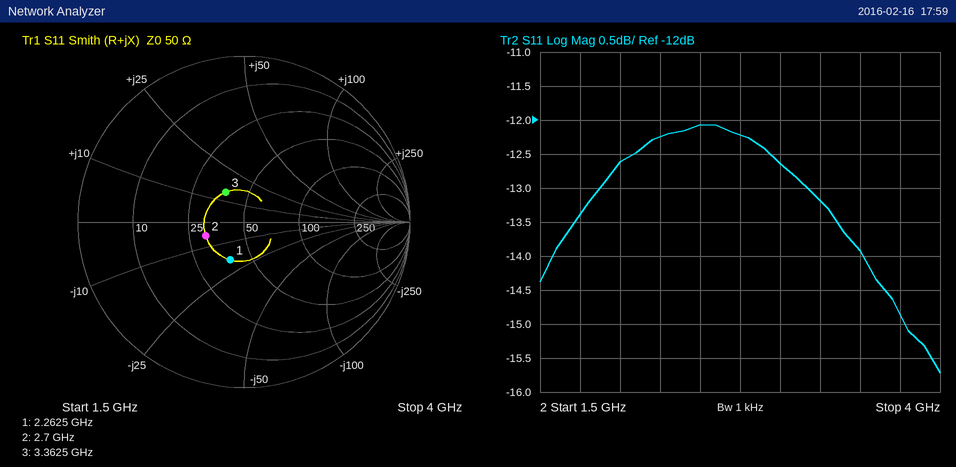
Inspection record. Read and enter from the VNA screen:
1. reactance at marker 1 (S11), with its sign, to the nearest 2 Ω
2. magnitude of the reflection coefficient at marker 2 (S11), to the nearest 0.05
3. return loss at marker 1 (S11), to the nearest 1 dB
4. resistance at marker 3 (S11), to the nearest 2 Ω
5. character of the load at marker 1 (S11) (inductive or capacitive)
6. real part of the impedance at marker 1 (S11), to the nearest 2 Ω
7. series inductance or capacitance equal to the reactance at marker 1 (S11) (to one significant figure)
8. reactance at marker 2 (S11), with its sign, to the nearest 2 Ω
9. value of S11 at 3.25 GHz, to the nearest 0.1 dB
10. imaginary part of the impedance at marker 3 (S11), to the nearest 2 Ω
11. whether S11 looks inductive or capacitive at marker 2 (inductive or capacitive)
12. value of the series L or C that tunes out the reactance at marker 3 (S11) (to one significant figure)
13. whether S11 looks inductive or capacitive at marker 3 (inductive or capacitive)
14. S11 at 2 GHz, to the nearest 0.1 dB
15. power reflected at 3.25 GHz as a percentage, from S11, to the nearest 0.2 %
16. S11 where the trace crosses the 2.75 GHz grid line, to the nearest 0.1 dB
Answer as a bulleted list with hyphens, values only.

- -18 Ω
- 0.25
- 12 dB
- 38 Ω
- capacitive
- 38 Ω
- 4 pF
- -6 Ω
- -13.2 dB
- +14 Ω
- capacitive
- 3 pF
- inductive
- -12.6 dB
- 4.8 %
- -12.2 dB
